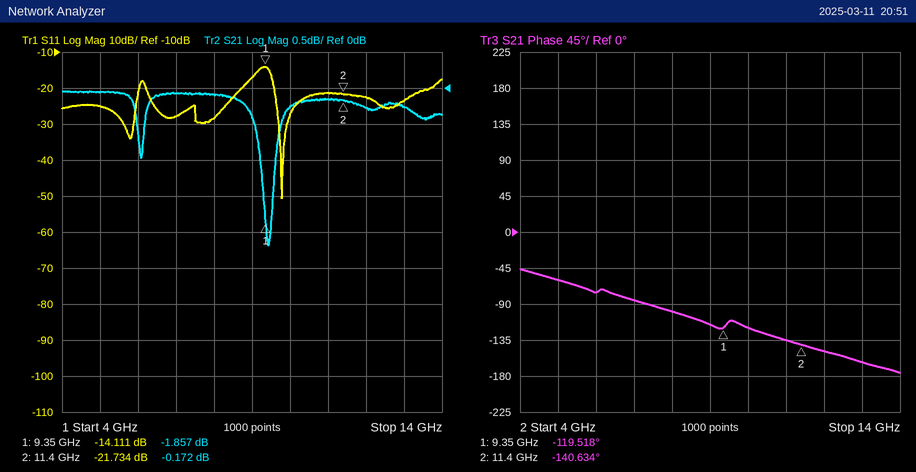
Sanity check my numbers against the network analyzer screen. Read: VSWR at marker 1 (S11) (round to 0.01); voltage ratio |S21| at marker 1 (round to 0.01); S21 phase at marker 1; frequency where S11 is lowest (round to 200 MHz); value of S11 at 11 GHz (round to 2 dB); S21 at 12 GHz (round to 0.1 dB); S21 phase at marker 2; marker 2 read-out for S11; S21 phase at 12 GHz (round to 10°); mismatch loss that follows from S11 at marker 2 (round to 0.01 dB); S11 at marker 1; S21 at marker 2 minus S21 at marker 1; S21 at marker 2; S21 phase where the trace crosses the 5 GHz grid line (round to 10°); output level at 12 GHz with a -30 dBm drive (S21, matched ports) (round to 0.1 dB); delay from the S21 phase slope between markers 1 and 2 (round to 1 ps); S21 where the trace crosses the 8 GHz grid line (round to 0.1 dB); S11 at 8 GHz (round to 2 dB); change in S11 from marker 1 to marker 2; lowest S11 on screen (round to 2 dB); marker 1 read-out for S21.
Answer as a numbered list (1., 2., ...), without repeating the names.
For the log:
1. 1.49
2. 0.81
3. -119.518°
4. 9.8 GHz
5. -22 dB
6. -0.3 dB
7. -140.634°
8. -21.734 dB
9. -150°
10. 0.03 dB
11. -14.111 dB
12. 1.685 dB
13. -0.172 dB
14. -60°
15. -30.3 dBm
16. 29 ps
17. -0.1 dB
18. -28 dB
19. -7.623 dB
20. -50 dB
21. -1.857 dB
